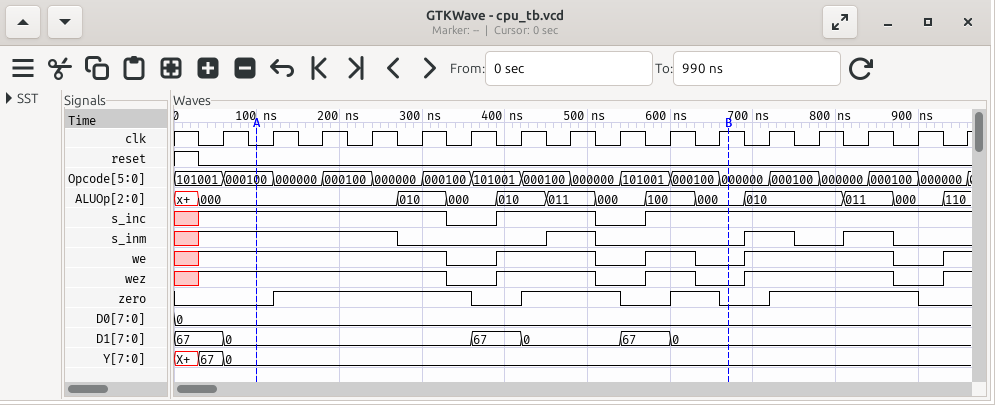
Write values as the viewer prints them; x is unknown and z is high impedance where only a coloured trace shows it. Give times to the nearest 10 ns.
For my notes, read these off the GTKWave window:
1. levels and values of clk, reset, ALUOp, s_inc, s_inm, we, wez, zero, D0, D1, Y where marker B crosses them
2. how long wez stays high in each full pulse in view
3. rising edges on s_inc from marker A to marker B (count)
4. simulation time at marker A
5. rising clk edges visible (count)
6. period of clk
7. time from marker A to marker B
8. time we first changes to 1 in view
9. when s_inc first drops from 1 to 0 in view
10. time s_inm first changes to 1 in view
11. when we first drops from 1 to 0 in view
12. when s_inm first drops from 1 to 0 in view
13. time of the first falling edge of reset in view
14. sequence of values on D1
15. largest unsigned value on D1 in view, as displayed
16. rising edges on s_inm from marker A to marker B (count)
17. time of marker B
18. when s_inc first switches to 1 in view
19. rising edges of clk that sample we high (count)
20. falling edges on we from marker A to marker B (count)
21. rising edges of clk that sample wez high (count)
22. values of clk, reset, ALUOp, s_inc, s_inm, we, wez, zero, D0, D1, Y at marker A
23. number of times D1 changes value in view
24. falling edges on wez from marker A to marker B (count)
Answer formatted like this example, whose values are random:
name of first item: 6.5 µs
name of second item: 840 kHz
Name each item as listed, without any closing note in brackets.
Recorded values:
levels and values of clk, reset, ALUOp, s_inc, s_inm, we, wez, zero, D0, D1, Y where marker B crosses them: clk=1, reset=0, ALUOp=000, s_inc=1, s_inm=0, we=0, wez=0, zero=0, D0=0, D1=0, Y=0
how long wez stays high in each full pulse in view: 120 ns, 60 ns, 180 ns
rising edges on s_inc from marker A to marker B: 2
simulation time at marker A: 100 ns
rising clk edges visible: 16
period of clk: 60 ns
time from marker A to marker B: 570 ns
time we first changes to 1 in view: 30 ns
when s_inc first drops from 1 to 0 in view: 330 ns
time s_inm first changes to 1 in view: 30 ns
when we first drops from 1 to 0 in view: 330 ns
when s_inm first drops from 1 to 0 in view: 270 ns
time of the first falling edge of reset in view: 30 ns
sequence of values on D1: 67, 0, 67, 0, 67, 0
largest unsigned value on D1 in view, as displayed: 67
rising edges on s_inm from marker A to marker B: 1
time of marker B: 670 ns
when s_inc first switches to 1 in view: 30 ns
rising edges of clk that sample we high: 12
falling edges on we from marker A to marker B: 3
rising edges of clk that sample wez high: 12
values of clk, reset, ALUOp, s_inc, s_inm, we, wez, zero, D0, D1, Y at marker A: clk=0, reset=0, ALUOp=000, s_inc=1, s_inm=1, we=1, wez=1, zero=0, D0=0, D1=0, Y=0
number of times D1 changes value in view: 5
falling edges on wez from marker A to marker B: 3
